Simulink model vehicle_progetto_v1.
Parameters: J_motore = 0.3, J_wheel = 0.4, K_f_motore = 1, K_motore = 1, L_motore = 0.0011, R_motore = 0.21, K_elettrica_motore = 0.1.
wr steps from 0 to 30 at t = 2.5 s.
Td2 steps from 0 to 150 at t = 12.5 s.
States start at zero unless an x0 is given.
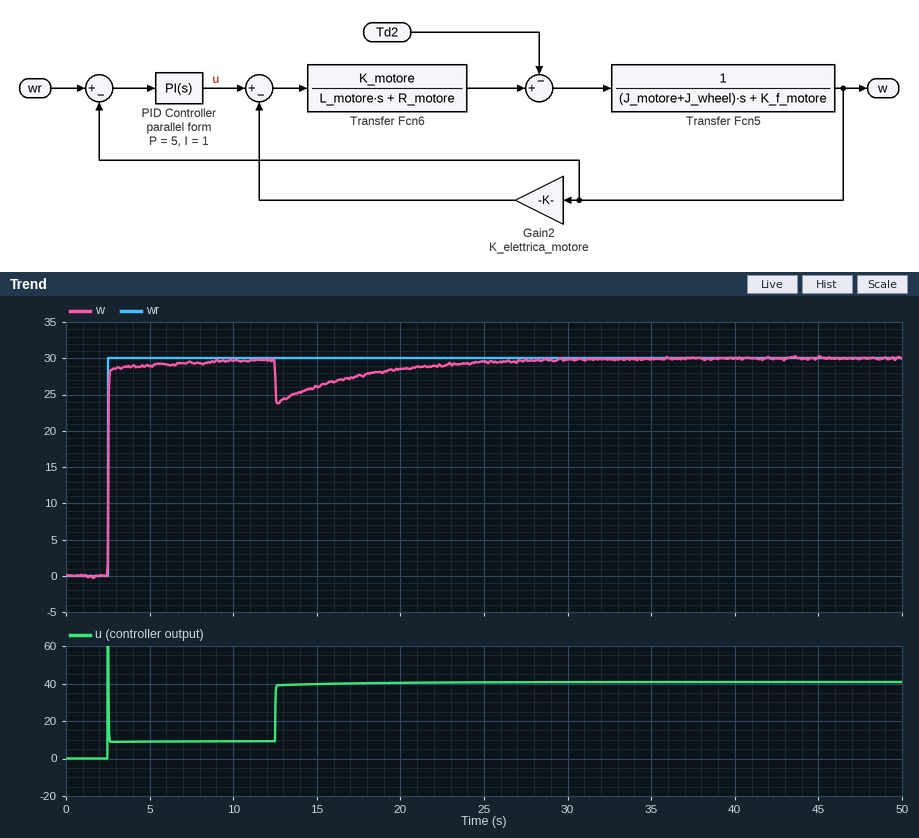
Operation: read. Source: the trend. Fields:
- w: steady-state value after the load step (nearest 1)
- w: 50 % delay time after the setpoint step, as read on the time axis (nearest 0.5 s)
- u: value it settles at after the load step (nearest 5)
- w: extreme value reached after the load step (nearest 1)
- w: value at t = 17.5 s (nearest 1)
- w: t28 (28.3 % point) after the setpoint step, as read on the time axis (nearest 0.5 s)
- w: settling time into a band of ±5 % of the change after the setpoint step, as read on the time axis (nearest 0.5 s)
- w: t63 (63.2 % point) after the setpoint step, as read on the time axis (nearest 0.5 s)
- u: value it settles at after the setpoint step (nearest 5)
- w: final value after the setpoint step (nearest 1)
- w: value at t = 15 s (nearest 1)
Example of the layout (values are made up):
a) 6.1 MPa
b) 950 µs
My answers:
a) 30
b) 2.5 s
c) 40
d) 24
e) 28
f) 2.5 s
g) 3.0 s
h) 2.5 s
i) 10
j) 30
k) 26
